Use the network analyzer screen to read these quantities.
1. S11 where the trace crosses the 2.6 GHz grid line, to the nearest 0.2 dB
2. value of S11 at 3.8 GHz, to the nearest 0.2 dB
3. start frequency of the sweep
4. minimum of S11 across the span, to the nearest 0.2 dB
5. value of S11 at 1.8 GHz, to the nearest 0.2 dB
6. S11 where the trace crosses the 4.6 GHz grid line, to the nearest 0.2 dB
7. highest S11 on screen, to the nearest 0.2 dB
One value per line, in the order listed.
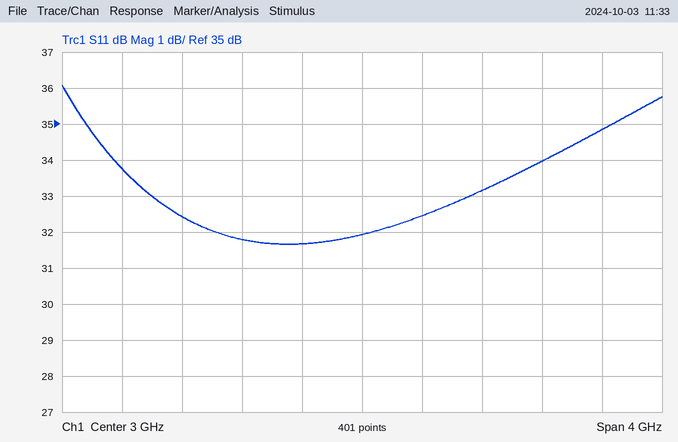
31.6 dB
33.2 dB
1 GHz
31.6 dB
32.4 dB
34.8 dB
36.0 dB
